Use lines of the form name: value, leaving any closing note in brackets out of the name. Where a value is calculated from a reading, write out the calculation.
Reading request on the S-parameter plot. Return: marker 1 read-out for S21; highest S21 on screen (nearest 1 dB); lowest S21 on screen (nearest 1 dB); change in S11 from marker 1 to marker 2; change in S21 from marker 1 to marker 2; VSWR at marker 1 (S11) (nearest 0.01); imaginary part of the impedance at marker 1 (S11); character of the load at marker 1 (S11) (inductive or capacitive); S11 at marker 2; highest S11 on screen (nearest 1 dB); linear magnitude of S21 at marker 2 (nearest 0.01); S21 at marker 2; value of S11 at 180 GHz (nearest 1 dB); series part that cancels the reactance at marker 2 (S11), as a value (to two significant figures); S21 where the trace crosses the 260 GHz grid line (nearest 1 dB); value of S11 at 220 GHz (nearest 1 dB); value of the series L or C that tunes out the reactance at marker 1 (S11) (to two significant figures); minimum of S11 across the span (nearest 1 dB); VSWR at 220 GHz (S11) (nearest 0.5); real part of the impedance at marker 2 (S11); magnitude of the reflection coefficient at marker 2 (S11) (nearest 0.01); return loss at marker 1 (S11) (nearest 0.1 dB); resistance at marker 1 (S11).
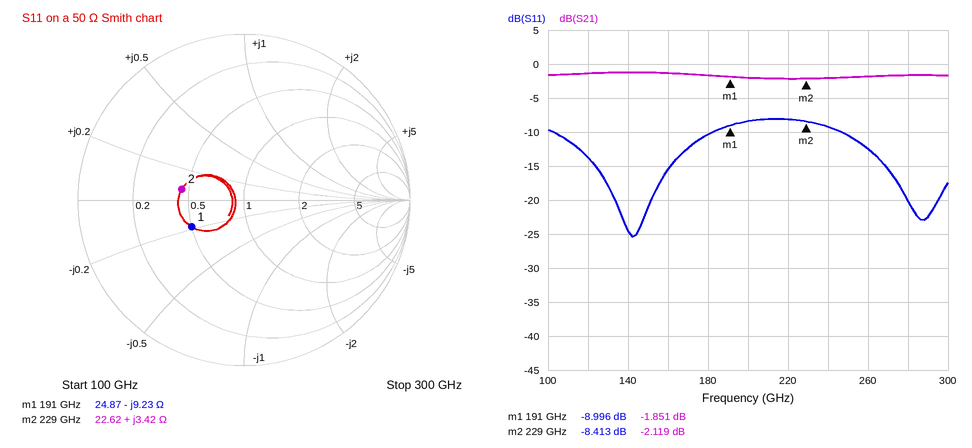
marker 1 read-out for S21: -1.851 dB
highest S21 on screen: -1 dB
lowest S21 on screen: -2 dB
change in S11 from marker 1 to marker 2: -8.413 − (-8.996) = 0.583 dB
change in S21 from marker 1 to marker 2: -2.119 − (-1.851) = -0.268 dB
VSWR at marker 1 (S11): (1 + 0.3550)/(1 − 0.3550) ≈ 2.10
imaginary part of the impedance at marker 1: -9.23 Ω
character of the load at marker 1 (S11): capacitive
S11 at marker 2: -8.413 dB
highest S11 on screen: -8 dB
linear magnitude of S21 at marker 2: 10^(-2.119/20) ≈ 0.78
S21 at marker 2: -2.119 dB
value of S11 at 180 GHz: -10 dB
series part that cancels the reactance at marker 2 (S11), as a value: C = 1/(2π × 229 GHz × 3.42 Ω) ≈ 203 fF, so 200 fF to two significant figures
S21 where the trace crosses the 260 GHz grid line: -2 dB
value of S11 at 220 GHz: -8 dB
value of the series L or C that tunes out the reactance at marker 1 (S11): L = 9.23 Ω/(2π × 191 GHz) ≈ 7.7 pH
minimum of S11 across the span: -25 dB
VSWR at 220 GHz (S11): |Γ| = 10^(-8/20) = 0.3981; VSWR = (1 + 0.3981)/(1 − 0.3981) ≈ 2.32, so 2.5 to the nearest 0.5
real part of the impedance at marker 2: 22.62 Ω
magnitude of the reflection coefficient at marker 2 (S11): 0.38
return loss at marker 1 (S11): 9.0 dB
resistance at marker 1: 24.87 Ω
